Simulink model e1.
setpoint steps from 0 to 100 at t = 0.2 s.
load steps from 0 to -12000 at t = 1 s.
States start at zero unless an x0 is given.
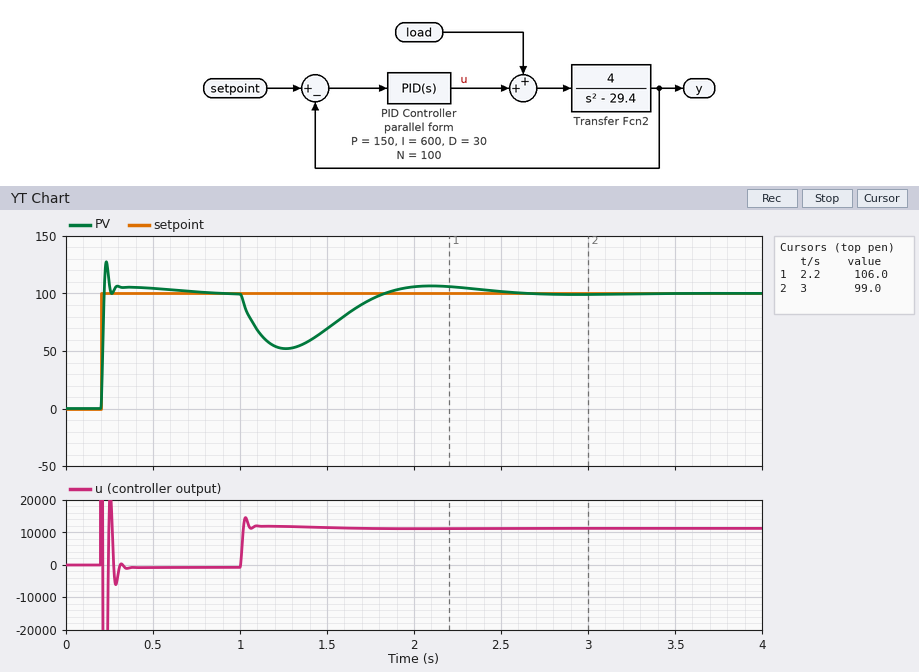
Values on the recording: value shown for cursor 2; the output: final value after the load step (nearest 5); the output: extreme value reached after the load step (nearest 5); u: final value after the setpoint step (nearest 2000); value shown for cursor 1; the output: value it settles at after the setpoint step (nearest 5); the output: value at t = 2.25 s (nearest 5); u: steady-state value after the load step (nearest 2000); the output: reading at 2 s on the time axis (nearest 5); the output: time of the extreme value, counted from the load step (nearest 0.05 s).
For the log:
99.0
100
50
0
106.0
100
105
12000
105
0.25 s
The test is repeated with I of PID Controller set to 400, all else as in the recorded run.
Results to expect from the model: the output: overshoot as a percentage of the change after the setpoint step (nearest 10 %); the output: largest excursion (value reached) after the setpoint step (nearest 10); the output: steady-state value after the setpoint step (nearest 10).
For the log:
30 %
130
100
